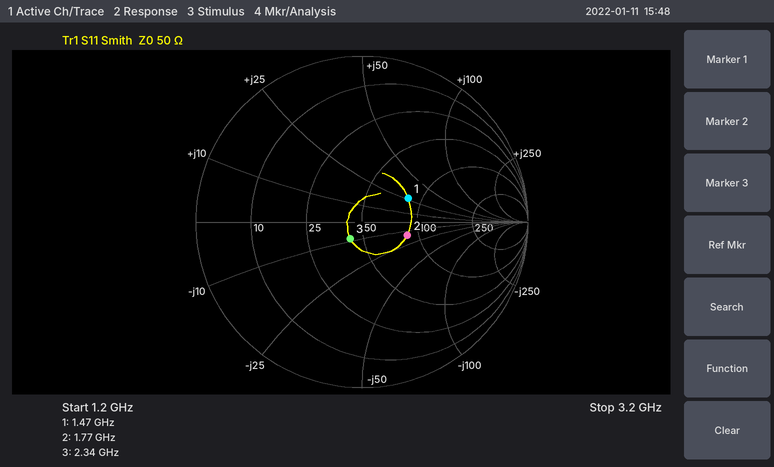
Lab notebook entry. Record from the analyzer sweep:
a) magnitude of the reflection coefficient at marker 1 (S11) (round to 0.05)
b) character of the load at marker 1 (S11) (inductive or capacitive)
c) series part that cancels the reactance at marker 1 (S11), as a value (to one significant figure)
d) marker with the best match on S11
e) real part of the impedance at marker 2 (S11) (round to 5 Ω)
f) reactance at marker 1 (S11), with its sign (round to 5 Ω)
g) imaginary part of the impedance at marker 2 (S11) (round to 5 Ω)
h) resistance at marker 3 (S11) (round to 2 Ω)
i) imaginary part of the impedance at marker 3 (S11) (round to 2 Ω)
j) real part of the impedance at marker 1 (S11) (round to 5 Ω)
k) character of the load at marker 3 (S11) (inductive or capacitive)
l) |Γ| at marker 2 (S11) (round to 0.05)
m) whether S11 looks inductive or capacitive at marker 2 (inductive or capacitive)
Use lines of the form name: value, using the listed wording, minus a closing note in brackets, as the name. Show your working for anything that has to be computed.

magnitude of the reflection coefficient at marker 1 (S11): 0.30
character of the load at marker 1 (S11): inductive
series part that cancels the reactance at marker 1 (S11), as a value: C = 1/(2π × 1.47 GHz × 25 Ω) ≈ 4 pF
marker with the best match on S11: marker 3
real part of the impedance at marker 2 (S11): 85 Ω
reactance at marker 1 (S11), with its sign: +25 Ω
imaginary part of the impedance at marker 2 (S11): -15 Ω
resistance at marker 3 (S11): 42 Ω
imaginary part of the impedance at marker 3 (S11): -8 Ω
real part of the impedance at marker 1 (S11): 85 Ω
character of the load at marker 3 (S11): capacitive
|Γ| at marker 2 (S11): 0.30
whether S11 looks inductive or capacitive at marker 2: capacitive
